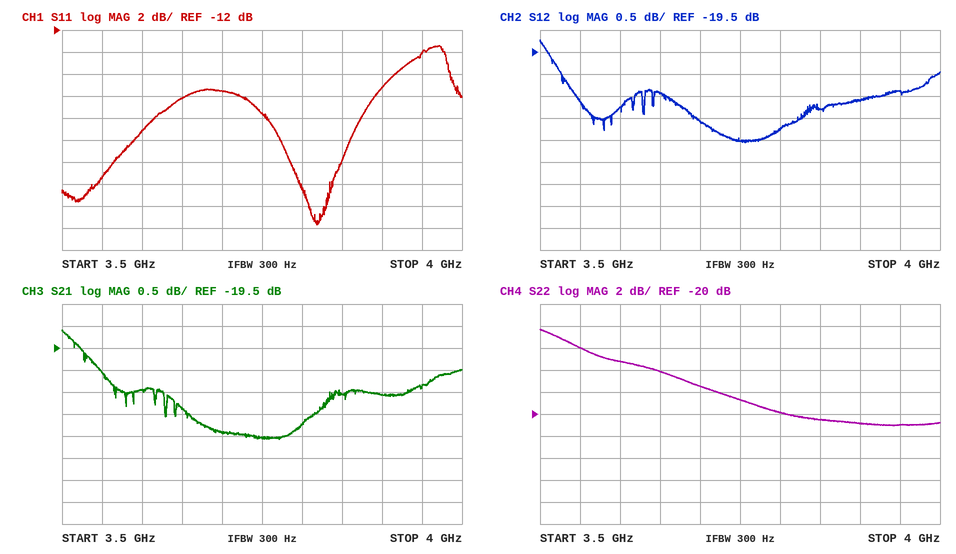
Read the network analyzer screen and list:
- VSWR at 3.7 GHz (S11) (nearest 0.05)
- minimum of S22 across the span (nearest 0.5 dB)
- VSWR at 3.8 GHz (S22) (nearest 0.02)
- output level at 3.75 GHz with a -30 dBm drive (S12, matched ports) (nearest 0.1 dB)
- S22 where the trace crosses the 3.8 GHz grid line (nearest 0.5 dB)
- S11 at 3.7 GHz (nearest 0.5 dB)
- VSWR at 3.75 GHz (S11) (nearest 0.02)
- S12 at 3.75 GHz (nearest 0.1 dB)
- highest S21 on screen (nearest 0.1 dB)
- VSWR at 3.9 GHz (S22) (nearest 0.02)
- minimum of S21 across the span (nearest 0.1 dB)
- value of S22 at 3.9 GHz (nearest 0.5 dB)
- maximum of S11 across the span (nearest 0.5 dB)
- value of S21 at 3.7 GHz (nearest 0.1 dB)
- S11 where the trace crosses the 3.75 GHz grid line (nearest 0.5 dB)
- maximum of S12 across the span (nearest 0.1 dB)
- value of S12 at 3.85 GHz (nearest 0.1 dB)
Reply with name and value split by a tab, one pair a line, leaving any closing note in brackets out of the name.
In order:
VSWR at 3.7 GHz (S11)	1.30
minimum of S22 across the span	-21.0 dB
VSWR at 3.8 GHz (S22)	1.22
output level at 3.75 GHz with a -30 dBm drive (S12, matched ports)	-51.5 dBm
S22 where the trace crosses the 3.8 GHz grid line	-20.0 dB
S11 at 3.7 GHz	-17.5 dB
VSWR at 3.75 GHz (S11)	1.24
S12 at 3.75 GHz	-21.5 dB
highest S21 on screen	-19.1 dB
VSWR at 3.9 GHz (S22)	1.20
minimum of S21 across the span	-21.6 dB
value of S22 at 3.9 GHz	-21.0 dB
maximum of S11 across the span	-13.5 dB
value of S21 at 3.7 GHz	-21.4 dB
S11 where the trace crosses the 3.75 GHz grid line	-19.5 dB
maximum of S12 across the span	-19.2 dB
value of S12 at 3.85 GHz	-20.8 dB
